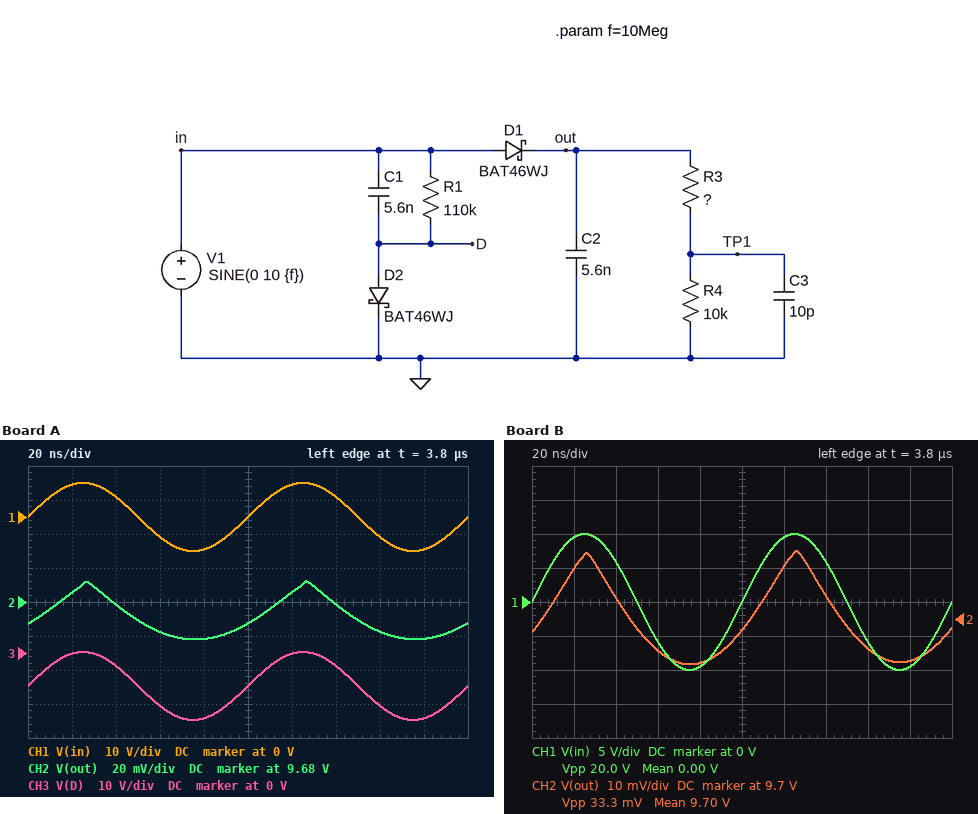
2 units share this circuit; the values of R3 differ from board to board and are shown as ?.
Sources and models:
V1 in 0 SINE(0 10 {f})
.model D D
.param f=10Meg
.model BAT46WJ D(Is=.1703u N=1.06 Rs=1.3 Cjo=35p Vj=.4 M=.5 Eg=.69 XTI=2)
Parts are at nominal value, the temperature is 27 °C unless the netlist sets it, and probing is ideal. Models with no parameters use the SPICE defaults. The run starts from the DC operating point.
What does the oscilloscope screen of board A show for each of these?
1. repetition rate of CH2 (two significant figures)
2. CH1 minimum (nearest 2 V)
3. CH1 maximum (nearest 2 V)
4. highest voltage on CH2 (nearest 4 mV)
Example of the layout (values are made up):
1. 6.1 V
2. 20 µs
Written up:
1. 10 MHz
2. -10 V
3. 10 V
4. 9.692 V
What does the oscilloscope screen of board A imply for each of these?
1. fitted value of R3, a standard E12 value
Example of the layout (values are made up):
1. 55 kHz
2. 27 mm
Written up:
1. 39 kΩ
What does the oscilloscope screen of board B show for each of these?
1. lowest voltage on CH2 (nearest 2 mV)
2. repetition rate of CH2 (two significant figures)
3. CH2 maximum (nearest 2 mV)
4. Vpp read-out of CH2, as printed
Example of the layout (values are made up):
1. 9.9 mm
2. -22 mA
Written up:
1. 9.686 V
2. 10 MHz
3. 9.720 V
4. 33.3 mV
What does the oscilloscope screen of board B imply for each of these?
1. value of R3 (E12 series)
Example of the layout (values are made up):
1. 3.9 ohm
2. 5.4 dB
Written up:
1. 180 kΩ
